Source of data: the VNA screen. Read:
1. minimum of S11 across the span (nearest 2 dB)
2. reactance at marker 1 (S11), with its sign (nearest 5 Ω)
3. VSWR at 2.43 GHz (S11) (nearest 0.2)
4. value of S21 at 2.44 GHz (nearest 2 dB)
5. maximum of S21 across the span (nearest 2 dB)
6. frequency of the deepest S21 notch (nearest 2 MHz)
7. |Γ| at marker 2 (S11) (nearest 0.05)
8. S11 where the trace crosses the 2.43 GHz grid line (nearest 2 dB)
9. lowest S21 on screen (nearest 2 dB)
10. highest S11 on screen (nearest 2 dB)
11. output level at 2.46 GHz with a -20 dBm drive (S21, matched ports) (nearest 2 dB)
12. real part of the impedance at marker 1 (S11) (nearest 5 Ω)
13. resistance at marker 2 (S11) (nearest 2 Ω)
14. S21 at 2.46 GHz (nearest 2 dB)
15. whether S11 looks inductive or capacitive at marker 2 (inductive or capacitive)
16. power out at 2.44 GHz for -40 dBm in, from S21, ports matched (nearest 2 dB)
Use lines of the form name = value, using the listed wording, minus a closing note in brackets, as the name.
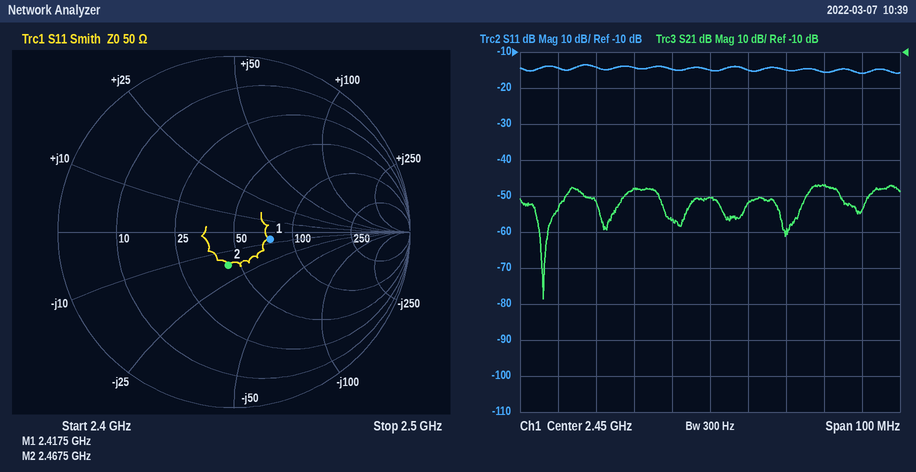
minimum of S11 across the span = -16 dB
reactance at marker 1 (S11), with its sign = -5 Ω
VSWR at 2.43 GHz (S11) = 1.4
value of S21 at 2.44 GHz = -56 dB
maximum of S21 across the span = -46 dB
frequency of the deepest S21 notch = 2.406 GHz
|Γ| at marker 2 (S11) = 0.20
S11 where the trace crosses the 2.43 GHz grid line = -14 dB
lowest S21 on screen = -78 dB
highest S11 on screen = -14 dB
output level at 2.46 GHz with a -20 dBm drive (S21, matched ports) = -72 dBm
real part of the impedance at marker 1 (S11) = 75 Ω
resistance at marker 2 (S11) = 44 Ω
S21 at 2.46 GHz = -52 dB
whether S11 looks inductive or capacitive at marker 2 = capacitive
power out at 2.44 GHz for -40 dBm in, from S21, ports matched = -96 dBm
